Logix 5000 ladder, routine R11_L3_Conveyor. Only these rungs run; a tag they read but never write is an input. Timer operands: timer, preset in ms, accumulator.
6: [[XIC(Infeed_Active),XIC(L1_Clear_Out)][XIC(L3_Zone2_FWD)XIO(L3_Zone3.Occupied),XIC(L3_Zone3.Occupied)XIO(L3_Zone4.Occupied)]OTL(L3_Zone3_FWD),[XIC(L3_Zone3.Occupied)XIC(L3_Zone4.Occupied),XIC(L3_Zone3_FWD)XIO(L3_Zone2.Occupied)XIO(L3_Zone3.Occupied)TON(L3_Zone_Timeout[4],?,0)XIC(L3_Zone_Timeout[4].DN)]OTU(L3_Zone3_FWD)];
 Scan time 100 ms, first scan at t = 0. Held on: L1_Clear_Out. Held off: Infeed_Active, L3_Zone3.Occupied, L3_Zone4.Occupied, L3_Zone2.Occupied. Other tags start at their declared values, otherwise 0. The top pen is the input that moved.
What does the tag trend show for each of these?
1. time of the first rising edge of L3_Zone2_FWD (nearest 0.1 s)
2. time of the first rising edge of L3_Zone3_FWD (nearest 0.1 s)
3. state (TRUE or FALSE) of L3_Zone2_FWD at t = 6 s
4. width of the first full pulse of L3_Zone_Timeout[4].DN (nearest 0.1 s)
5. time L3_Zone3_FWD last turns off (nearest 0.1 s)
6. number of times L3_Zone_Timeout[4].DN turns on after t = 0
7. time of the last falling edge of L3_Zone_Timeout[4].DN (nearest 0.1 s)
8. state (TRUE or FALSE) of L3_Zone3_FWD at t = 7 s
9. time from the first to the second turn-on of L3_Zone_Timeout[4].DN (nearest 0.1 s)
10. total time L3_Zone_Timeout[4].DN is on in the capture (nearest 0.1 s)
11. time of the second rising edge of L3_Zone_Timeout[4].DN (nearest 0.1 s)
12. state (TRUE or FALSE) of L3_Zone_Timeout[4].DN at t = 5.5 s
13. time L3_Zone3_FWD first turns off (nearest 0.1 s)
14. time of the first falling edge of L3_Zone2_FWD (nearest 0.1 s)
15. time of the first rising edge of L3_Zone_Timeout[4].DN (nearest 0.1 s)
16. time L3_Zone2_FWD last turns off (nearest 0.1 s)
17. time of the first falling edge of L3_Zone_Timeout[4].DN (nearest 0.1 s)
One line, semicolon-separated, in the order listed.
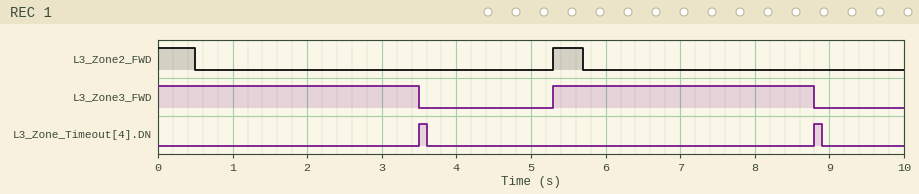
5.3 s; 5.3 s; FALSE; 0.1 s; 8.8 s; 2; 8.9 s; TRUE; 5.3 s; 0.2 s; 8.8 s; FALSE; 3.5 s; 0.5 s; 3.5 s; 5.7 s; 3.6 s
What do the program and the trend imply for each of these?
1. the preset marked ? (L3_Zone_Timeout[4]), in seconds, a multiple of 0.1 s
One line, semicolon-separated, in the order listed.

3.5 s
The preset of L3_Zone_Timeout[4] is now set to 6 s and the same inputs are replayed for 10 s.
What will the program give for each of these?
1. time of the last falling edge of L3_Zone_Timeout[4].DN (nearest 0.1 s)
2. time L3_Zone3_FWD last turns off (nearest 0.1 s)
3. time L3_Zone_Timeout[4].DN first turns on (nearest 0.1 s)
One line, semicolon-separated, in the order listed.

6.1 s; 6.0 s; 6.0 s
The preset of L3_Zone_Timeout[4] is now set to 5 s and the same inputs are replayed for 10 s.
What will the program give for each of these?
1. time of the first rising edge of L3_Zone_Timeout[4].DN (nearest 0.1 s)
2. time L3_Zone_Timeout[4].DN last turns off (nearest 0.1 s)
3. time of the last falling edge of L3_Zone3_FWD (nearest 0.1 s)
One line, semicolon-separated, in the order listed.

5.0 s; 5.1 s; 5.0 s
